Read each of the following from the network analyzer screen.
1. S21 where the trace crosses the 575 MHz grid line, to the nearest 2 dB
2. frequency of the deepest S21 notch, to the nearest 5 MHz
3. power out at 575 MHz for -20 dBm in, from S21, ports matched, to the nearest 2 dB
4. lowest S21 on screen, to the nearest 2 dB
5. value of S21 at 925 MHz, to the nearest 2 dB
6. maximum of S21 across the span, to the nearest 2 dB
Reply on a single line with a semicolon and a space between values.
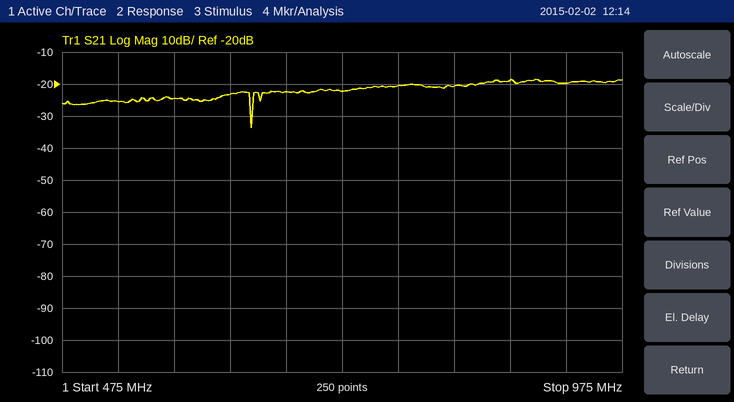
-24 dB; 645 MHz; -44 dBm; -34 dB; -20 dB; -18 dB
